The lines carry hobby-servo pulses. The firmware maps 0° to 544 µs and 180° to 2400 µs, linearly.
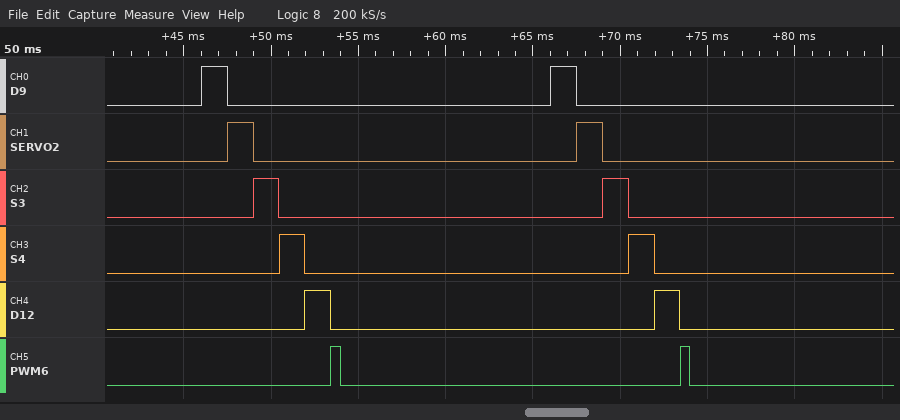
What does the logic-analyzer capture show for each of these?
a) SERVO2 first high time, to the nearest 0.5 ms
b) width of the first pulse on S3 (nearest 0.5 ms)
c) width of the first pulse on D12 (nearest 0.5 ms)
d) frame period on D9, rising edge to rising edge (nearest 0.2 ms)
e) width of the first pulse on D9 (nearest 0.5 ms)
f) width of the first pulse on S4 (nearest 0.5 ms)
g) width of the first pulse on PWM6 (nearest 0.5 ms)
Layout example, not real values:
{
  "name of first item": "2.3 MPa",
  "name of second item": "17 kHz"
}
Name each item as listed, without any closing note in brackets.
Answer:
{
  "SERVO2 first high time, to the nearest 0.5 ms": "1.5 ms",
  "width of the first pulse on S3": "1.5 ms",
  "width of the first pulse on D12": "1.5 ms",
  "frame period on D9, rising edge to rising edge": "20.0 ms",
  "width of the first pulse on D9": "1.5 ms",
  "width of the first pulse on S4": "1.5 ms",
  "width of the first pulse on PWM6": "0.5 ms"
}
